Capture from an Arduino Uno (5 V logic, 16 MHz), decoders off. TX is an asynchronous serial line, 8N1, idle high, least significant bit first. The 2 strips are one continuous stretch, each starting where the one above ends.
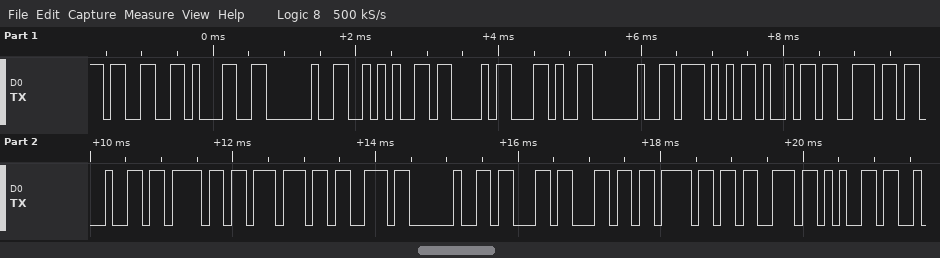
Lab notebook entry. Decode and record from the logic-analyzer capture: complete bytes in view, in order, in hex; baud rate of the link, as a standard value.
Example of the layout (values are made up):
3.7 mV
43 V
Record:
33 31 20 2A 43 2C 20 57 69 6E 64 6F 77 73 20 63 6C 6F 73 65
9600 baud
